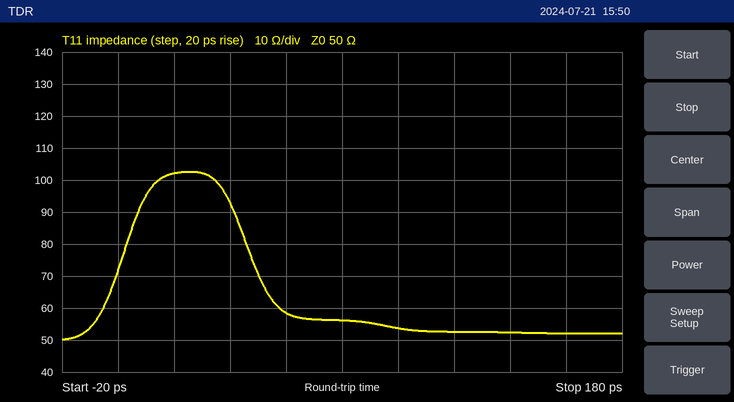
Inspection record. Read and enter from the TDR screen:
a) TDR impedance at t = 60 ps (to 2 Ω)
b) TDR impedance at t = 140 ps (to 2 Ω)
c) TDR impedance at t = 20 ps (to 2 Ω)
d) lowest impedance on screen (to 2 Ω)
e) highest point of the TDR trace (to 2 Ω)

58 Ω
52 Ω
102 Ω
50 Ω
102 Ω
